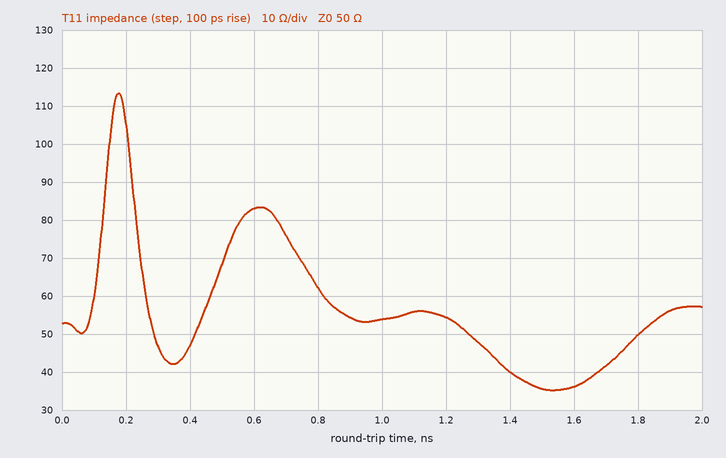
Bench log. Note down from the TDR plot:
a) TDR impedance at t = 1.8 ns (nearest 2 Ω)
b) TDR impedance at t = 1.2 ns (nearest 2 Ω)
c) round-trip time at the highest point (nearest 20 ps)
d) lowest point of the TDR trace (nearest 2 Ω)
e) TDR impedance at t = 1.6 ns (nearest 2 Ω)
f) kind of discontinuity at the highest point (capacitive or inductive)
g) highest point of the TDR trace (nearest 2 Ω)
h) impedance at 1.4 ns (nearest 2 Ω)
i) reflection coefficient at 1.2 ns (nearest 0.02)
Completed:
50 Ω
54 Ω
180 ps
36 Ω
36 Ω
inductive
114 Ω
40 Ω
+0.04
